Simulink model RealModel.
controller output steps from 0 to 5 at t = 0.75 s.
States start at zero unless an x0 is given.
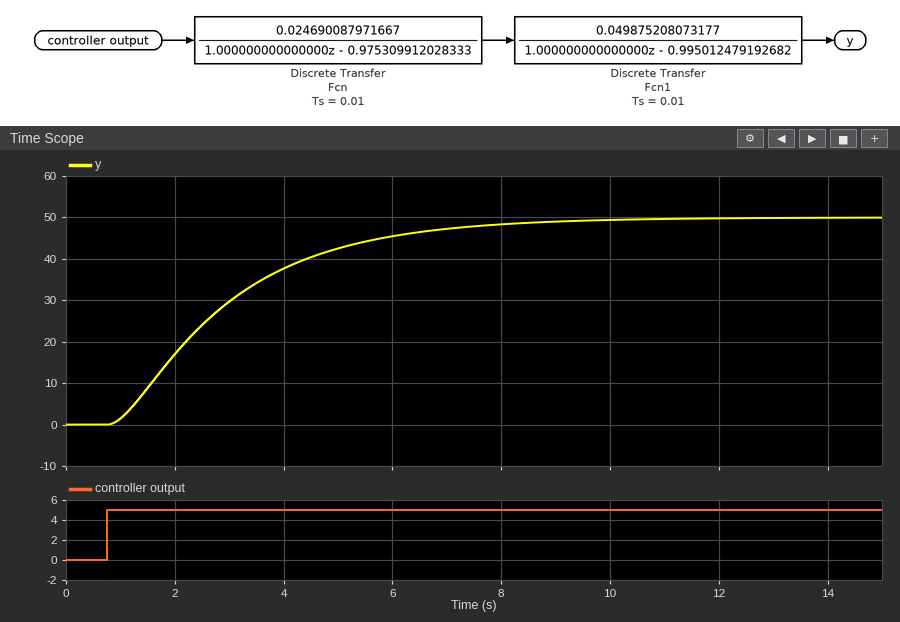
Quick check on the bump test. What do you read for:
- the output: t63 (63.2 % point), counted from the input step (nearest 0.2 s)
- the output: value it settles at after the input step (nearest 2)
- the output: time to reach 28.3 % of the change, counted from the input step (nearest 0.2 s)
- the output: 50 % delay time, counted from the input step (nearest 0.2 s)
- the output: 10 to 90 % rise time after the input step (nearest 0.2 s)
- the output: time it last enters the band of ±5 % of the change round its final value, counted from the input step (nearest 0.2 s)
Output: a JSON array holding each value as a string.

["2.4 s", "50", "1.0 s", "1.8 s", "4.6 s", "6.4 s"]
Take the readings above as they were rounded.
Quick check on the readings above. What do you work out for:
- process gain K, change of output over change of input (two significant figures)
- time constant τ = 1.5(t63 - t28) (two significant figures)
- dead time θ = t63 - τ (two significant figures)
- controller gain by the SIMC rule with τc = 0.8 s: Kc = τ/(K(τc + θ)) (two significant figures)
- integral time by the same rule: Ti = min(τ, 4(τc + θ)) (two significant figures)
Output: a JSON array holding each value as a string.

["10", "2.1 s", "0.30 s", "0.19", "2.1 s"]
